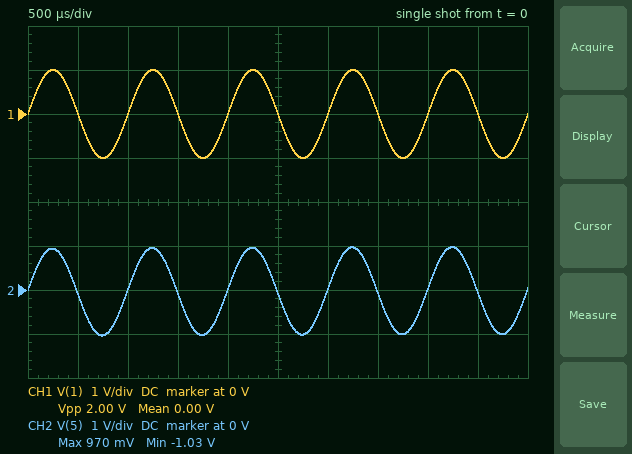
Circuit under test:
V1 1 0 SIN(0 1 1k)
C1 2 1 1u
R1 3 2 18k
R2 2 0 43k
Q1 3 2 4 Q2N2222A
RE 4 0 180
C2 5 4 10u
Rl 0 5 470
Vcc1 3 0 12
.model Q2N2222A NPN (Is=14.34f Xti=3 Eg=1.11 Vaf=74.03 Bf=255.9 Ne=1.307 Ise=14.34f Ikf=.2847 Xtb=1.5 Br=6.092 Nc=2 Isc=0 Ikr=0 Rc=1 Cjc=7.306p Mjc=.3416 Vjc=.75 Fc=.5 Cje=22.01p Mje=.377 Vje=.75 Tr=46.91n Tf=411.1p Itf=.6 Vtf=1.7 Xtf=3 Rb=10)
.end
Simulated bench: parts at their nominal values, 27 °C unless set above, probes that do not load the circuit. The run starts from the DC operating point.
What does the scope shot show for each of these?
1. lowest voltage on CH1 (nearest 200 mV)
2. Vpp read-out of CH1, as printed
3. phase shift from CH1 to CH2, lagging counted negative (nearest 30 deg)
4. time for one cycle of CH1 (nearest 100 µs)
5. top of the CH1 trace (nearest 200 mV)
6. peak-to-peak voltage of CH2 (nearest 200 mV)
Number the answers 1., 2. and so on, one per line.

1. -1.0 V
2. 2.00 V
3. 0 deg
4. 1.0 ms
5. 1.0 V
6. 2.0 V
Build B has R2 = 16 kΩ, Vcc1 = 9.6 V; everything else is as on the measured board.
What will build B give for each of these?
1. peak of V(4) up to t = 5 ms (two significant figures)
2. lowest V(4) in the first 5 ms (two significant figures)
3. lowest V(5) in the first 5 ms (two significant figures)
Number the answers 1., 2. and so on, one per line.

1. 4.0 V
2. 2.0 V
3. -1.0 V
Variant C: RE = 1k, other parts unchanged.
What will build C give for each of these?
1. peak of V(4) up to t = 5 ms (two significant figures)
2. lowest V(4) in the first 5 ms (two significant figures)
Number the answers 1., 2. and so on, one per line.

1. 8.2 V
2. 6.3 V
